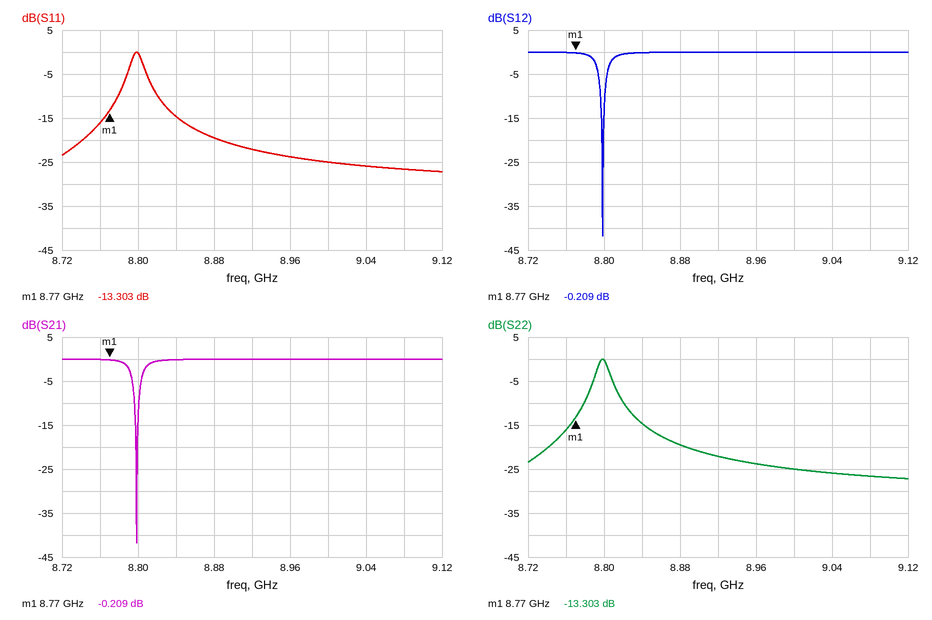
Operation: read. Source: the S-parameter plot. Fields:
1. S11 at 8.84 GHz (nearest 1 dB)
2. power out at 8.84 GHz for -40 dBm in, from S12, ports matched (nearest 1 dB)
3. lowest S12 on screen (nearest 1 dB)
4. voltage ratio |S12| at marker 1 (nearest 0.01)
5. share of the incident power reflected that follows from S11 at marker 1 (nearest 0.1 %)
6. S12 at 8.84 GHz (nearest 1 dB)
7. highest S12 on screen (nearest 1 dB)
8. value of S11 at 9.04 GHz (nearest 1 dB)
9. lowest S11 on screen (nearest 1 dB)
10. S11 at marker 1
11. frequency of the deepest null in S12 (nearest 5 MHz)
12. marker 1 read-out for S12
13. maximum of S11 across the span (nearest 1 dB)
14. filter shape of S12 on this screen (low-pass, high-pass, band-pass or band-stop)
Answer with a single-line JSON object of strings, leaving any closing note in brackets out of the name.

{"S11 at 8.84 GHz": "-15 dB", "power out at 8.84 GHz for -40 dBm in, from S12, ports matched": "-40 dBm", "lowest S12 on screen": "-42 dB", "voltage ratio |S12| at marker 1": "0.98", "share of the incident power reflected that follows from S11 at marker 1": "4.7 %", "S12 at 8.84 GHz": "0 dB", "highest S12 on screen": "0 dB", "value of S11 at 9.04 GHz": "-26 dB", "lowest S11 on screen": "-27 dB", "S11 at marker 1": "-13.303 dB", "frequency of the deepest null in S12": "8.800 GHz", "marker 1 read-out for S12": "-0.209 dB", "maximum of S11 across the span": "0 dB", "filter shape of S12 on this screen": "band-stop"}
